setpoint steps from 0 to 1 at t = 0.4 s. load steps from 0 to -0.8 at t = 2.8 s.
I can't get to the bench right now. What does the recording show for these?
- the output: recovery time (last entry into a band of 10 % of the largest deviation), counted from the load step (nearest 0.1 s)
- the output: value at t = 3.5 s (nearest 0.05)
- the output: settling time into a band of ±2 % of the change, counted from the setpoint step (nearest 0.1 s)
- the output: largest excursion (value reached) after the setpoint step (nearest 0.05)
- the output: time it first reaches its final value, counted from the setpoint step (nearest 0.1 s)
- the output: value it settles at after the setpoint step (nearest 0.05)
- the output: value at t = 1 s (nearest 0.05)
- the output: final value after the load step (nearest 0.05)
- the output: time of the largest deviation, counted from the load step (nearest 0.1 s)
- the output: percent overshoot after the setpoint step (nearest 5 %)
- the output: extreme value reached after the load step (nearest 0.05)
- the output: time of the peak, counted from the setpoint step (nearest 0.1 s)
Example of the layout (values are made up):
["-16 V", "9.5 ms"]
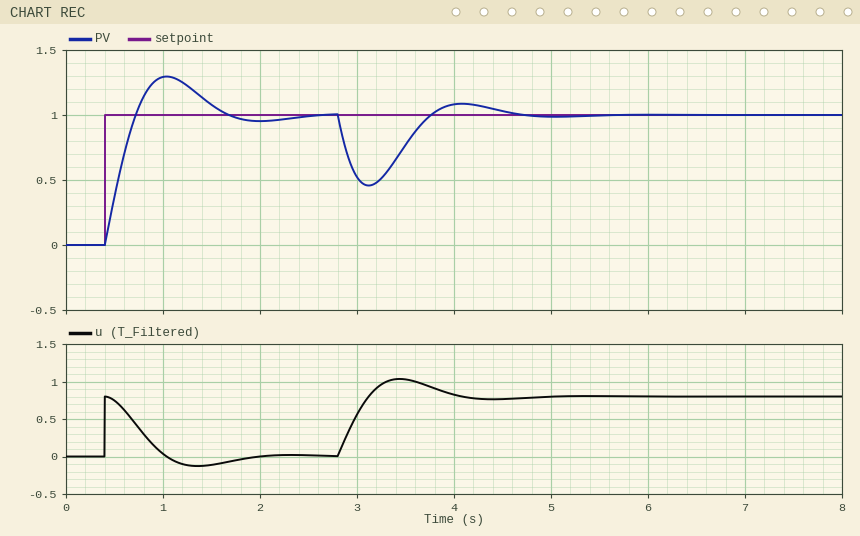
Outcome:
["1.6 s", "0.75", "2.0 s", "1.30", "0.3 s", "1.00", "1.30", "1.00", "0.3 s", "30 %", "0.45", "0.6 s"]
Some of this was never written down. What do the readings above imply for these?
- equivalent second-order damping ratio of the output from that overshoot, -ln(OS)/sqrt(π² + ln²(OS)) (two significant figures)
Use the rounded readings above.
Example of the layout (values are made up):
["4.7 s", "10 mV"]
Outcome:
["0.36"]
